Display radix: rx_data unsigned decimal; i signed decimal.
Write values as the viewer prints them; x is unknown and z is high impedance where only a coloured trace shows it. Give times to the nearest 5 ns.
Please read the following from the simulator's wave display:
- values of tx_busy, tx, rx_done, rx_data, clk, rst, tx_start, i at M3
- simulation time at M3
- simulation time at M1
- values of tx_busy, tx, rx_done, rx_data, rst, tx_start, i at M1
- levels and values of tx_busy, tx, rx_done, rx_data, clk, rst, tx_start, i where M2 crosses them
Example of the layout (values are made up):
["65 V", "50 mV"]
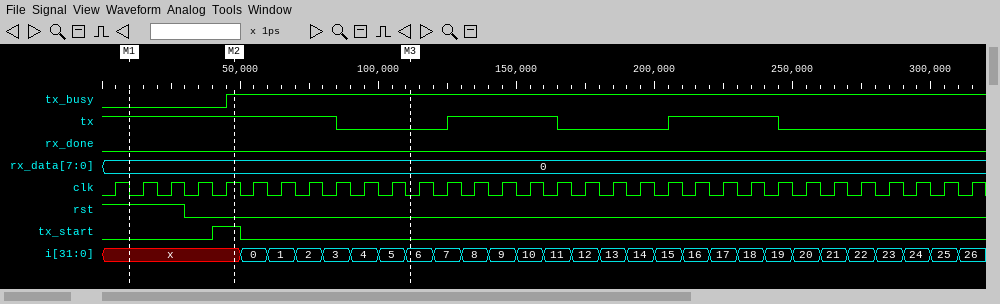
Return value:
["tx_busy=1, tx=0, rx_done=0, rx_data=0, clk=0, rst=0, tx_start=0, i=6", "110 ns", "10 ns", "tx_busy=0, tx=1, rx_done=0, rx_data=0, rst=1, tx_start=0, i=x", "tx_busy=1, tx=1, rx_done=0, rx_data=0, clk=1, rst=0, tx_start=1, i=x"]
